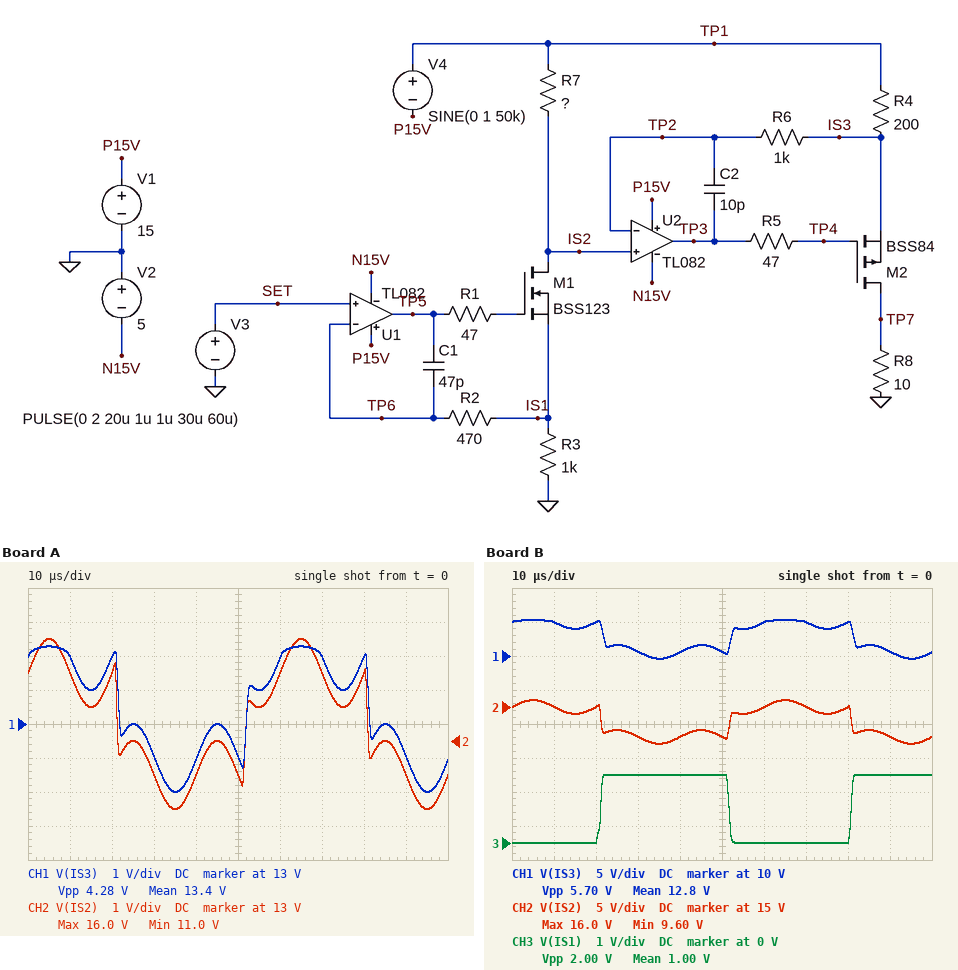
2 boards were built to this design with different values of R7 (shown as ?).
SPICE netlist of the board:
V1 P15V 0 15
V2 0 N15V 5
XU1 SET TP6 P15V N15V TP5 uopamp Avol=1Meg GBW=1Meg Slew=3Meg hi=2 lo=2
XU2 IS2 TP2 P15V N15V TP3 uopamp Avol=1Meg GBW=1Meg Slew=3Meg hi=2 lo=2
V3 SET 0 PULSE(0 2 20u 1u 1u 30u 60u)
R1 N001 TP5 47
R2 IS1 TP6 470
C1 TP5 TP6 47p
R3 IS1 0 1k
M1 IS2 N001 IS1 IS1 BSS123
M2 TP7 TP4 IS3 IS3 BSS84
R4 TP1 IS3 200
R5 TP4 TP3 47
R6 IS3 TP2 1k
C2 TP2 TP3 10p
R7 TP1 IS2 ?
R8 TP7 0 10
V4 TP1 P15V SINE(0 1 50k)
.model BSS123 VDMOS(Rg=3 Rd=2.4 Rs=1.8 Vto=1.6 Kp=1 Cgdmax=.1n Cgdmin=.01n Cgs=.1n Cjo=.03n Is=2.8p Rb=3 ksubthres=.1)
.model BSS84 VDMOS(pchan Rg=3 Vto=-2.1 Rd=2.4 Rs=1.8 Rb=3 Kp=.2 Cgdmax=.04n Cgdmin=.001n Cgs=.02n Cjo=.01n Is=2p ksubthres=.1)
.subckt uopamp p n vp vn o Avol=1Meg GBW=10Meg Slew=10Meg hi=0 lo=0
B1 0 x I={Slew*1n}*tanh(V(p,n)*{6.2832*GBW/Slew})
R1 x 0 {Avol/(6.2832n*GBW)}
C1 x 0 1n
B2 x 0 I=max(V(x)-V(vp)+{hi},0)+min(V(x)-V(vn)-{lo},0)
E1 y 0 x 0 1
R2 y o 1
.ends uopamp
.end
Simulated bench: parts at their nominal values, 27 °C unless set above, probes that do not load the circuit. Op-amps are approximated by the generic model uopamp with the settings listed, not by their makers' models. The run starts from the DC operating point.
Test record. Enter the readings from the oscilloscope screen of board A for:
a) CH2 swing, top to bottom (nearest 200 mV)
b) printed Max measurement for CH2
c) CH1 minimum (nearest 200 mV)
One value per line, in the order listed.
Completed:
5.0 V
16.0 V
11.0 V
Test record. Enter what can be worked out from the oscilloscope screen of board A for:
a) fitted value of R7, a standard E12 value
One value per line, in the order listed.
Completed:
1.5 kΩ
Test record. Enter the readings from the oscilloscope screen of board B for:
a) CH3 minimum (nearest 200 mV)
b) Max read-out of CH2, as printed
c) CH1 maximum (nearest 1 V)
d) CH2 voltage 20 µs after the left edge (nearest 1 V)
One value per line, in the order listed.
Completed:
0 V
16.0 V
15 V
15 V
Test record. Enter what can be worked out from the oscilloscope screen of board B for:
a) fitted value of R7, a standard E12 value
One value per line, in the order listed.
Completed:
2.2 kΩ
